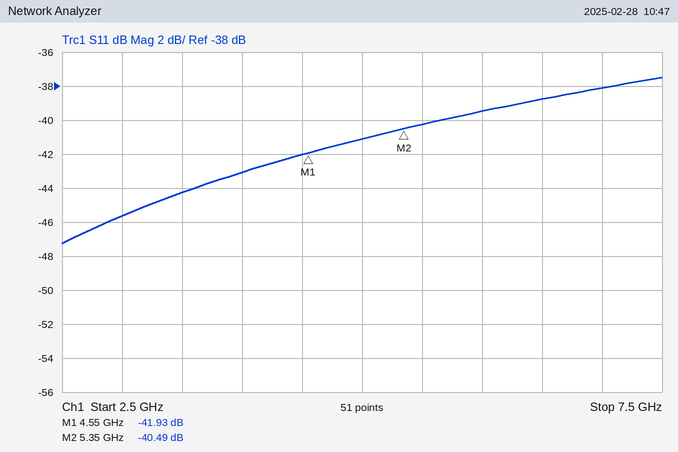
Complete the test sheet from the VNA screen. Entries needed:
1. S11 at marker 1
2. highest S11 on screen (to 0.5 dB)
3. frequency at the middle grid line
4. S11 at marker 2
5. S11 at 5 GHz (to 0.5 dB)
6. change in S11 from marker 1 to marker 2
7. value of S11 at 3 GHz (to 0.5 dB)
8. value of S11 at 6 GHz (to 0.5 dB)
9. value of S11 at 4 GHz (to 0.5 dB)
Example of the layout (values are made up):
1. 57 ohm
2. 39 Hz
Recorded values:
1. -41.93 dB
2. -37.5 dB
3. 5 GHz
4. -40.49 dB
5. -41.0 dB
6. 1.44 dB
7. -45.5 dB
8. -39.5 dB
9. -43.0 dB
